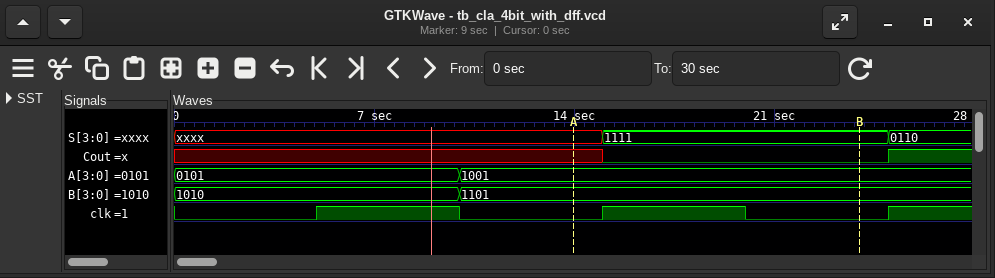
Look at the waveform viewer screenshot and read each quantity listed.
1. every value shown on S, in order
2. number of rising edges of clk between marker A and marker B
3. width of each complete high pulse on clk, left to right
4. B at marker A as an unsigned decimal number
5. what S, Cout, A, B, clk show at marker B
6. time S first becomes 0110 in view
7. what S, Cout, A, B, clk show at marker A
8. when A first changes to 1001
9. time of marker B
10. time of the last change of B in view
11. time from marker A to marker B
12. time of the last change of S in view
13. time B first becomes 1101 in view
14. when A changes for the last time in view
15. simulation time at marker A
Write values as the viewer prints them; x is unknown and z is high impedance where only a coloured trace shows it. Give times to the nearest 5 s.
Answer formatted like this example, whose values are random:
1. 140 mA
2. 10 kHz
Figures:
1. xxxx, 1111, 0110
2. 1
3. 5 s, 5 s
4. 13
5. S=1111, Cout=0, A=1001, B=1101, clk=0
6. 25 s
7. S=xxxx, Cout=x, A=1001, B=1101, clk=0
8. 10 s
9. 25 s
10. 10 s
11. 10 s
12. 25 s
13. 10 s
14. 10 s
15. 15 s
